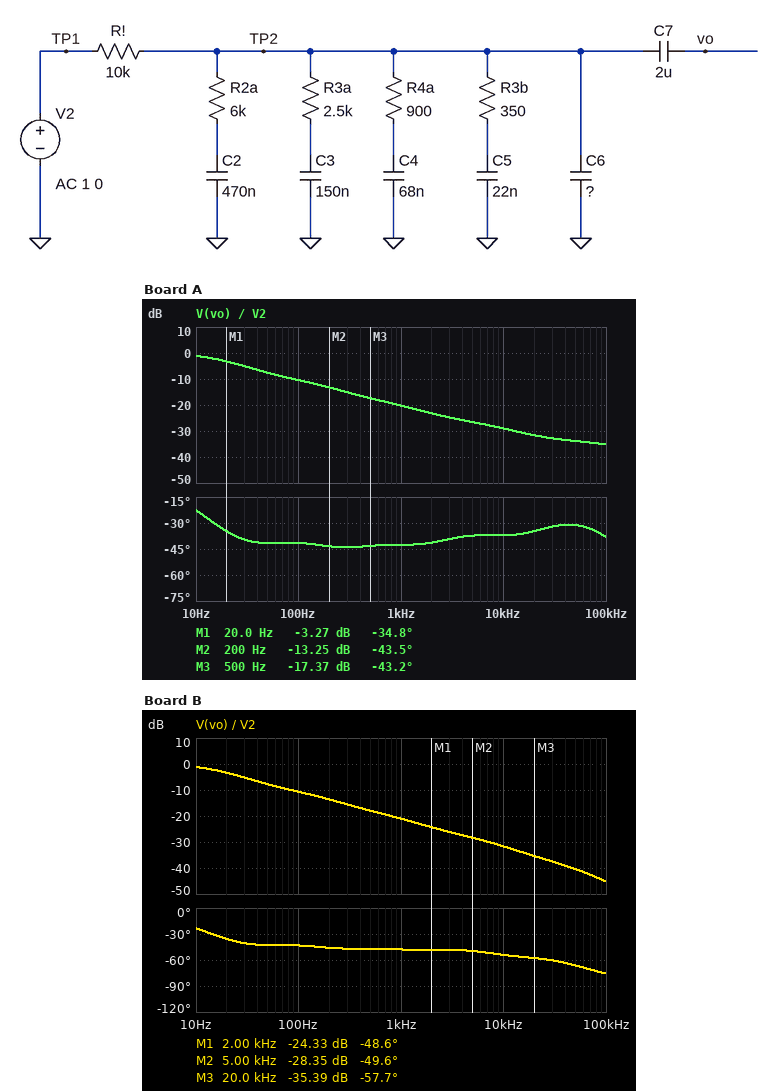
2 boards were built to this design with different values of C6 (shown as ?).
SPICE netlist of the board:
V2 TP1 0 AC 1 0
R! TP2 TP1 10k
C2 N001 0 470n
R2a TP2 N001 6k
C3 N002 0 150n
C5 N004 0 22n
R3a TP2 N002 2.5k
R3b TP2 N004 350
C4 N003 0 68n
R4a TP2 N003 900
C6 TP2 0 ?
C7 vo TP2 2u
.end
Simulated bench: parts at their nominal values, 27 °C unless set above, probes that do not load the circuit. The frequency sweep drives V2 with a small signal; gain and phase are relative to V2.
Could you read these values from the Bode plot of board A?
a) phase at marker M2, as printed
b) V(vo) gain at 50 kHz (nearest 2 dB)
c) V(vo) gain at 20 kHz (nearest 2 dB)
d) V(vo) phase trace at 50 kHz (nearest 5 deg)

-43.5 deg
-34 dB
-32 dB
-30 deg
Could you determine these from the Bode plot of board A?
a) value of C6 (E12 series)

4.7 nF
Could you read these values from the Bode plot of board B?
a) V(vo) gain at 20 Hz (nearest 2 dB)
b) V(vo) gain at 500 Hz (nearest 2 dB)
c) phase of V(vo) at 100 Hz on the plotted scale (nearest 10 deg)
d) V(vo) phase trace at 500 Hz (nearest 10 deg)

-4 dB
-18 dB
-40 deg
-50 deg
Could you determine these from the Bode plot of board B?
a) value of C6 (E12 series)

27 nF
